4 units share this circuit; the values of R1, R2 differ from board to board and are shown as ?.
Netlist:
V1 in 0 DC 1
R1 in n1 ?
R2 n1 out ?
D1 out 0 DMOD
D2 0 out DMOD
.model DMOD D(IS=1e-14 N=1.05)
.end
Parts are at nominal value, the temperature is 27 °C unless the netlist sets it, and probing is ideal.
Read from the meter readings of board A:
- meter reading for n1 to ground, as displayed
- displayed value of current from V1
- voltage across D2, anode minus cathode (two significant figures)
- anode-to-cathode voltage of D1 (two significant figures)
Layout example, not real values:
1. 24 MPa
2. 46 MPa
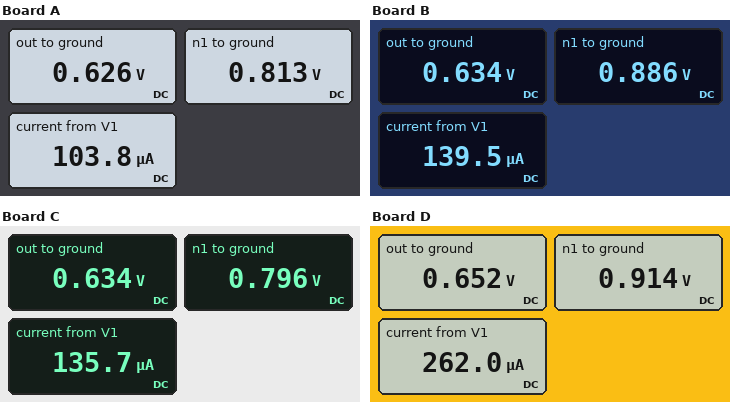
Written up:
1. 0.813 V
2. 103.8 µA
3. -630 mV
4. 630 mV
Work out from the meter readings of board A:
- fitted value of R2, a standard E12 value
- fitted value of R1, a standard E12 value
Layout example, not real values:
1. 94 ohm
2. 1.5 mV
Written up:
1. 1.8 kΩ
2. 1.8 kΩ
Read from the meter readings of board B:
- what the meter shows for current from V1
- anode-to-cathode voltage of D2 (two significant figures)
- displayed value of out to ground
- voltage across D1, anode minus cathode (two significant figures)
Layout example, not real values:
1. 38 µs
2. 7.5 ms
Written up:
1. 139.5 µA
2. -630 mV
3. 0.634 V
4. 630 mV
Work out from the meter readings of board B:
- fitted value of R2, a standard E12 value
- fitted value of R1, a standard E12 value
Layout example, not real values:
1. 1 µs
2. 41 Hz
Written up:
1. 1.8 kΩ
2. 820 Ω
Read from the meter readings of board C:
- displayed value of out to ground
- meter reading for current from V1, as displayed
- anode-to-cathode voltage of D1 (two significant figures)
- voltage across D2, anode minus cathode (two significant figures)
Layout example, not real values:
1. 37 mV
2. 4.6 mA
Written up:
1. 0.634 V
2. 135.7 µA
3. 630 mV
4. -630 mV
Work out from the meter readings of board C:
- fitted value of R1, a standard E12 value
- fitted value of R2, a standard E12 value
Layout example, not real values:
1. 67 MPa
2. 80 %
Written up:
1. 1.5 kΩ
2. 1.2 kΩ
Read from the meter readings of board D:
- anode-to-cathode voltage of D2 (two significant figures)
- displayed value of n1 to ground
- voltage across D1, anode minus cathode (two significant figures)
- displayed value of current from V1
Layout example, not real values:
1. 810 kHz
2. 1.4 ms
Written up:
1. -650 mV
2. 0.914 V
3. 650 mV
4. 262.0 µA
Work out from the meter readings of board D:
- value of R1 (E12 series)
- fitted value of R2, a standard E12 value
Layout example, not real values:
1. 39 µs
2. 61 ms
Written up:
1. 330 Ω
2. 1 kΩ
